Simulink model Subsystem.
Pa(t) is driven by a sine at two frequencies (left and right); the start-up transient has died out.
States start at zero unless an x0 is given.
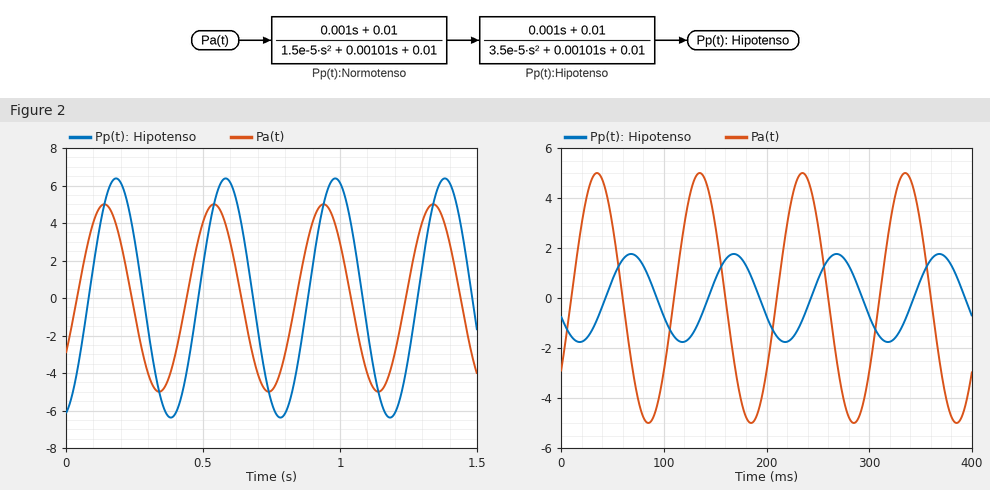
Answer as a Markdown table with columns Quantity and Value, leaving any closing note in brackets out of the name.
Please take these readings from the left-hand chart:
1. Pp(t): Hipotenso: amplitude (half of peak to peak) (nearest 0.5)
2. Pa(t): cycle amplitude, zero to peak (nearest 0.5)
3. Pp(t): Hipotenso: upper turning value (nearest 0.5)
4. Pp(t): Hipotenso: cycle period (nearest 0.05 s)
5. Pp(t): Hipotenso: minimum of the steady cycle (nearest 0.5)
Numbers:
| Quantity | Value |
|---|---|
| Pp(t): Hipotenso: amplitude (half of peak to peak) | 6.5 |
| Pa(t): cycle amplitude, zero to peak | 5.0 |
| Pp(t): Hipotenso: upper turning value | 6.5 |
| Pp(t): Hipotenso: cycle period | 0.40 s |
| Pp(t): Hipotenso: minimum of the steady cycle | -6.5 |
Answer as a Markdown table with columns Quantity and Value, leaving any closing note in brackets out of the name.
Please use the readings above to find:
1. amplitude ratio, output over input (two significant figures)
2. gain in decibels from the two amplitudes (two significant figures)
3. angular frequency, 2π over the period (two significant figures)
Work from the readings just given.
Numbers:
| Quantity | Value |
|---|---|
| amplitude ratio, output over input | 1.3 |
| gain in decibels from the two amplitudes | 2.3 dB |
| angular frequency, 2π over the period | 16 rad/s |
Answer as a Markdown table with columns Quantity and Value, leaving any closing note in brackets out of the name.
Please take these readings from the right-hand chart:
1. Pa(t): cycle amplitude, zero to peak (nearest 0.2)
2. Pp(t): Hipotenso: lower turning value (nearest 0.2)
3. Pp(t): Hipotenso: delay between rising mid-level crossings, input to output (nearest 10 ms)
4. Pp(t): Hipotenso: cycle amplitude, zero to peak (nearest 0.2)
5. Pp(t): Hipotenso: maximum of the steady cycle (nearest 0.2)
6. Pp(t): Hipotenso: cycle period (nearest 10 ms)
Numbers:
| Quantity | Value |
|---|---|
| Pa(t): cycle amplitude, zero to peak | 5.0 |
| Pp(t): Hipotenso: lower turning value | -1.8 |
| Pp(t): Hipotenso: delay between rising mid-level crossings, input to output | 30 ms |
| Pp(t): Hipotenso: cycle amplitude, zero to peak | 1.8 |
| Pp(t): Hipotenso: maximum of the steady cycle | 1.8 |
| Pp(t): Hipotenso: cycle period | 100 ms |
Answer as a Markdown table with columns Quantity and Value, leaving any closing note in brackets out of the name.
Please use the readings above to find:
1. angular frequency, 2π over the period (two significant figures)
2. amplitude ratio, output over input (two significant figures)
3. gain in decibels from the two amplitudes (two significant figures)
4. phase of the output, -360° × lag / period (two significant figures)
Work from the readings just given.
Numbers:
| Quantity | Value |
|---|---|
| angular frequency, 2π over the period | 0.063 rad/ms |
| amplitude ratio, output over input | 0.36 |
| gain in decibels from the two amplitudes | -8.9 dB |
| phase of the output, -360° × lag / period | -110° |
